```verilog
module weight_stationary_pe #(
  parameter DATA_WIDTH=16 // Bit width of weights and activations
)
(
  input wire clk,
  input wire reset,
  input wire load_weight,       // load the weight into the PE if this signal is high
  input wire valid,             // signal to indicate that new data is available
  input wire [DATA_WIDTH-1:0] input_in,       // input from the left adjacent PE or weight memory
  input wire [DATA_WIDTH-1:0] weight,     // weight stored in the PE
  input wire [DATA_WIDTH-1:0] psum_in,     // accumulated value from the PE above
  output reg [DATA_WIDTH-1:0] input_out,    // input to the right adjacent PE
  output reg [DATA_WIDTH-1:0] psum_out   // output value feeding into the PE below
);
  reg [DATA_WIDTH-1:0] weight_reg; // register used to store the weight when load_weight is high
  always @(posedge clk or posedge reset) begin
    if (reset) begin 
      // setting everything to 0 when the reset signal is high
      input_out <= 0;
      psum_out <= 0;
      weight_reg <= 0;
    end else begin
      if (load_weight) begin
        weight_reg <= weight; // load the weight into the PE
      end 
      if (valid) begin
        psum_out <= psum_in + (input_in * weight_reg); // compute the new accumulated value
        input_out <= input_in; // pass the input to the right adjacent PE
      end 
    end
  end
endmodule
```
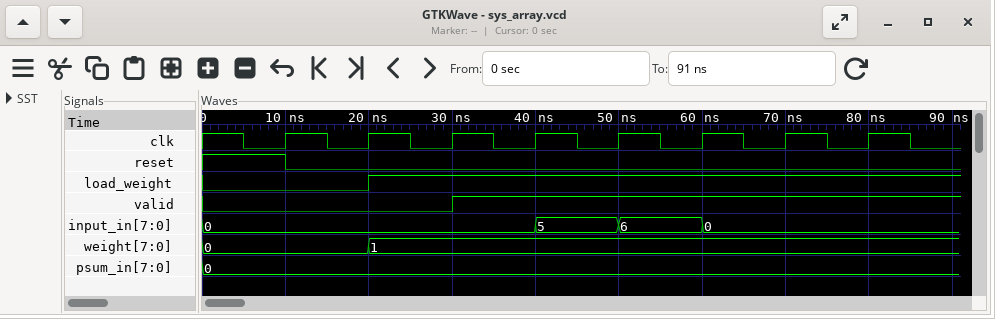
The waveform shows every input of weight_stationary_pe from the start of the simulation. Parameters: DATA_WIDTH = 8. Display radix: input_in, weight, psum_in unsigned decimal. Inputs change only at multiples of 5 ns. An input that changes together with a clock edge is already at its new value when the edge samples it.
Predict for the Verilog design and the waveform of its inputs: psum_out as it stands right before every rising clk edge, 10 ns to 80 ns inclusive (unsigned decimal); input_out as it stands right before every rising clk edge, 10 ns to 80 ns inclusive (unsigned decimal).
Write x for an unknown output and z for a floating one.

0, 0, 0, 0, 5, 6, 0, 0
0, 0, 0, 0, 5, 6, 0, 0
